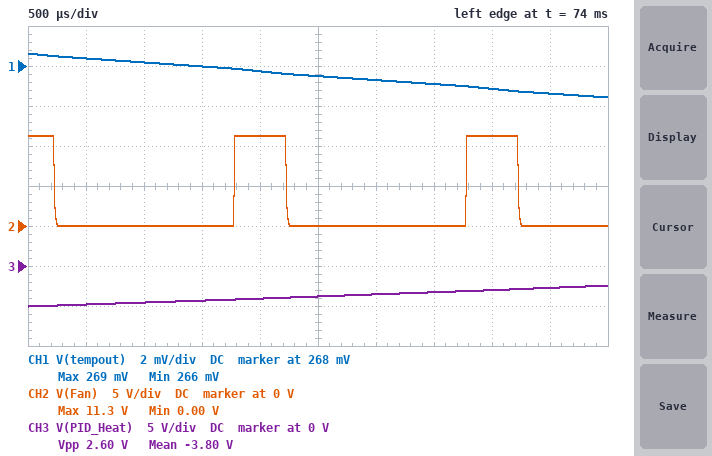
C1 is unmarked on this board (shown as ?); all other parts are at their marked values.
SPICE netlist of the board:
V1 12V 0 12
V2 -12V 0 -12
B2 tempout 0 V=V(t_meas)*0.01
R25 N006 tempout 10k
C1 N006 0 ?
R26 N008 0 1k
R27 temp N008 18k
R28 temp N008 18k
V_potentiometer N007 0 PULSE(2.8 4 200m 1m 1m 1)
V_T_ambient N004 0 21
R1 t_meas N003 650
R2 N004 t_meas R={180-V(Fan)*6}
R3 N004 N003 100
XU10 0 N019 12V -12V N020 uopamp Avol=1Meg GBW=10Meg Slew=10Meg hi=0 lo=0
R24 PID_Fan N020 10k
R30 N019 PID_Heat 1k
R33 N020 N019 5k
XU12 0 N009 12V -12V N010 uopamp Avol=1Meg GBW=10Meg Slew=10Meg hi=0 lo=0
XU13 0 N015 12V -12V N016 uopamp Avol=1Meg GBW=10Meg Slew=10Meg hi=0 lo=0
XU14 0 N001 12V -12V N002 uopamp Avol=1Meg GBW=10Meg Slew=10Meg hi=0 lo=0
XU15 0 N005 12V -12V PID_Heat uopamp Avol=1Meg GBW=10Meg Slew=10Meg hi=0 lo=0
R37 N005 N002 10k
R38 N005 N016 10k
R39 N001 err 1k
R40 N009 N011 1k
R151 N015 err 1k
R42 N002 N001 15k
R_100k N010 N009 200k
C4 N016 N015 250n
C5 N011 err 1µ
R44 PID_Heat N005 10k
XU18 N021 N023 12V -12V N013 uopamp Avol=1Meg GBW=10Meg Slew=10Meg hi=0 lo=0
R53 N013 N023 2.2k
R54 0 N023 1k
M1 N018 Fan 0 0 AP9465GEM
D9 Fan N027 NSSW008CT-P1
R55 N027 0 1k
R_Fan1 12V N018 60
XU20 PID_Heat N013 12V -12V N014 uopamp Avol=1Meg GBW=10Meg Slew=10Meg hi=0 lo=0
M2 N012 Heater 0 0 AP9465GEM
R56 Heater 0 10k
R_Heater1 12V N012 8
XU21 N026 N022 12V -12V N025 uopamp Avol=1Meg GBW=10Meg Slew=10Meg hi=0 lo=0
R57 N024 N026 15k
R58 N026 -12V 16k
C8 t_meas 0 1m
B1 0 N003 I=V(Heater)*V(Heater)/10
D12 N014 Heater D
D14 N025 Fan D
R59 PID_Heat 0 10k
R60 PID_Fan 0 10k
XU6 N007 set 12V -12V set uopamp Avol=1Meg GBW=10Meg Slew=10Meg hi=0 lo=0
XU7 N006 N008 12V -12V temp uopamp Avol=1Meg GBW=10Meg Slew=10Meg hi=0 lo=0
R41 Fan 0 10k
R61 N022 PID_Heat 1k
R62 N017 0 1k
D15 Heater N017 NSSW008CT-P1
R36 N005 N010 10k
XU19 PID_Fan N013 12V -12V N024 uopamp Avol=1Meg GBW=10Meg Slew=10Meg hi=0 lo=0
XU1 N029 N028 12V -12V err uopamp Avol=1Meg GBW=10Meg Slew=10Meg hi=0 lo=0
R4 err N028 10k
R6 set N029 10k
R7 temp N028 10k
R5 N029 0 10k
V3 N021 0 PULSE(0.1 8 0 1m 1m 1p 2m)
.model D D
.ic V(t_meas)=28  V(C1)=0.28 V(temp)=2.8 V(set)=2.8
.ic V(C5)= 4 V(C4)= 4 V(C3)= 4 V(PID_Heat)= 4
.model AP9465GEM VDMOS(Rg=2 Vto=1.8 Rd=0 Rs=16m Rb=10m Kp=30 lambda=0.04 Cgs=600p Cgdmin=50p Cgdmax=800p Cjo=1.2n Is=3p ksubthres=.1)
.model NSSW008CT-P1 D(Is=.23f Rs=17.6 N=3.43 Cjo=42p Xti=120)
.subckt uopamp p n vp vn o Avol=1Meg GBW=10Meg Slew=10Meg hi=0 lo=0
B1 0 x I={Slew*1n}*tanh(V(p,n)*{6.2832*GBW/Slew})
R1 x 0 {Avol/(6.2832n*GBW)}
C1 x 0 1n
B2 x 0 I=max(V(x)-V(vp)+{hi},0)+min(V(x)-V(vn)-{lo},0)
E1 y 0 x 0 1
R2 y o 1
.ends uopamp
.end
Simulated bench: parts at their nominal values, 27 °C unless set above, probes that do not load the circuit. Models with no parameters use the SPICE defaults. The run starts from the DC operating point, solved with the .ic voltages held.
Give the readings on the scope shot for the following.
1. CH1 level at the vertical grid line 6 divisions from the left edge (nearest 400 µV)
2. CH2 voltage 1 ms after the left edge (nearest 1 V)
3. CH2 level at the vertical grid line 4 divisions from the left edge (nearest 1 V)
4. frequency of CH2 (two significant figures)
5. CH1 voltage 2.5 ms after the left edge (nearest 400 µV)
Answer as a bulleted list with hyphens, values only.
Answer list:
- 267.2 mV
- 0 V
- 11 V
- 500 Hz
- 267.6 mV
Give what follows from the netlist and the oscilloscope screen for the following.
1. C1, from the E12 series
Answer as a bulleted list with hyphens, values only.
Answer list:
- 220 nF
